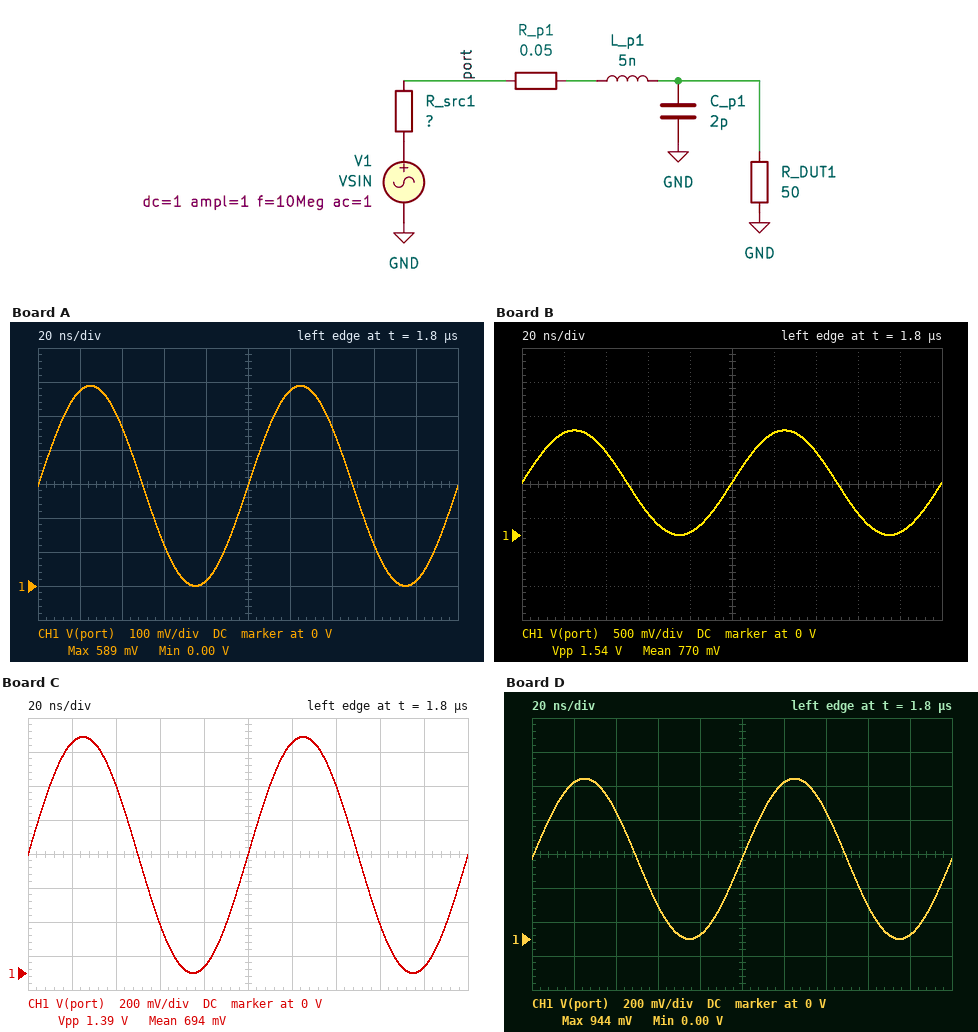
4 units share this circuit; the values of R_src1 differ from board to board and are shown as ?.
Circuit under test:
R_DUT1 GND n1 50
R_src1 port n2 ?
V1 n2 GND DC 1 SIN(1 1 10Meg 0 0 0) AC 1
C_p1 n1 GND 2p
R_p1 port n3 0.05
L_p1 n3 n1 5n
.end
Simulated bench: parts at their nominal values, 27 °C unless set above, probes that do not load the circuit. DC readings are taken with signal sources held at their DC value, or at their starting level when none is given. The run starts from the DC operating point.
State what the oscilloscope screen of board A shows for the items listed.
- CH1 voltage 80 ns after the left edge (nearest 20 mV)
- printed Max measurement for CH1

20 mV
589 mV
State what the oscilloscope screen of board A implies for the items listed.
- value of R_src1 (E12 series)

120 Ω
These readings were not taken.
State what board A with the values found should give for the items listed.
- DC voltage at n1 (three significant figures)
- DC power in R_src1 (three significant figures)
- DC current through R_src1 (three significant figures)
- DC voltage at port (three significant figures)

294 mV
4.15 mW
5.88 mA
294 mV
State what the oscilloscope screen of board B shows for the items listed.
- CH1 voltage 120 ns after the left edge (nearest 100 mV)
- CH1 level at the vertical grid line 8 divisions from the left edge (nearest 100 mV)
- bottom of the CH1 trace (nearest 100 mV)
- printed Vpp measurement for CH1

1.5 V
300 mV
0 V
1.54 V
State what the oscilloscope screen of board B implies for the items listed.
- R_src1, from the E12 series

15 Ω
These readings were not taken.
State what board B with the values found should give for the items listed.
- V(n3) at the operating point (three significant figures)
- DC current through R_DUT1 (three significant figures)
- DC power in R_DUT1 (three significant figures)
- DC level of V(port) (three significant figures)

769 mV
15.4 mA
11.8 mW
769 mV
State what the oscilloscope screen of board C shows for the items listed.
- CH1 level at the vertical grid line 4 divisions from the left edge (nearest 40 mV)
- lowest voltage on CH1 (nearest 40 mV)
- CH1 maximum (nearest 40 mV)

40 mV
0 V
1.40 V
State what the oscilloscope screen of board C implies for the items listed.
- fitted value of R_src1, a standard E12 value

22 Ω
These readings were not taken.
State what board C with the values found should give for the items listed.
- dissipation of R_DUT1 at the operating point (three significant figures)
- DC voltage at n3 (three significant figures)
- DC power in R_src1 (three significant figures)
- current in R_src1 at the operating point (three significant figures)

9.63 mW
694 mV
4.24 mW
13.9 mA
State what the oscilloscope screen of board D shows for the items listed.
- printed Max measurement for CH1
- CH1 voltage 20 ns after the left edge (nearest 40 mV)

944 mV
920 mV
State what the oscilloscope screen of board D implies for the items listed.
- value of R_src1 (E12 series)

56 Ω
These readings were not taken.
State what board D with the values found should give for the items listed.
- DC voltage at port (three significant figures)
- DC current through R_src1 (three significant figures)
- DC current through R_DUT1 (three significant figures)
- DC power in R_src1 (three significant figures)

472 mV
9.43 mA
9.43 mA
4.98 mW
